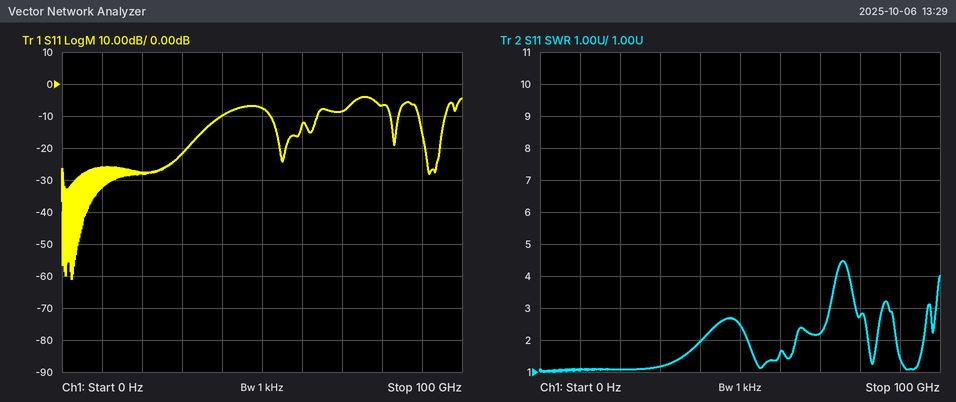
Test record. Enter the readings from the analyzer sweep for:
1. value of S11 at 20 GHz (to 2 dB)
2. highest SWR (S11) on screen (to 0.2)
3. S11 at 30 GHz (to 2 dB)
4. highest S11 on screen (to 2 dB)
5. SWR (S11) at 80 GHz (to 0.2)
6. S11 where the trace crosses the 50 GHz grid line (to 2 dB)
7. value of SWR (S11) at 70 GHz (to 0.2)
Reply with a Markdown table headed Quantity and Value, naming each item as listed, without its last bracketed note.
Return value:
| Quantity | Value |
|---|---|
| value of S11 at 20 GHz | -28 dB |
| highest SWR (S11) on screen | 4.4 |
| S11 at 30 GHz | -22 dB |
| highest S11 on screen | -4 dB |
| SWR (S11) at 80 GHz | 2.8 |
| S11 where the trace crosses the 50 GHz grid line | -8 dB |
| value of SWR (S11) at 70 GHz | 2.2 |
